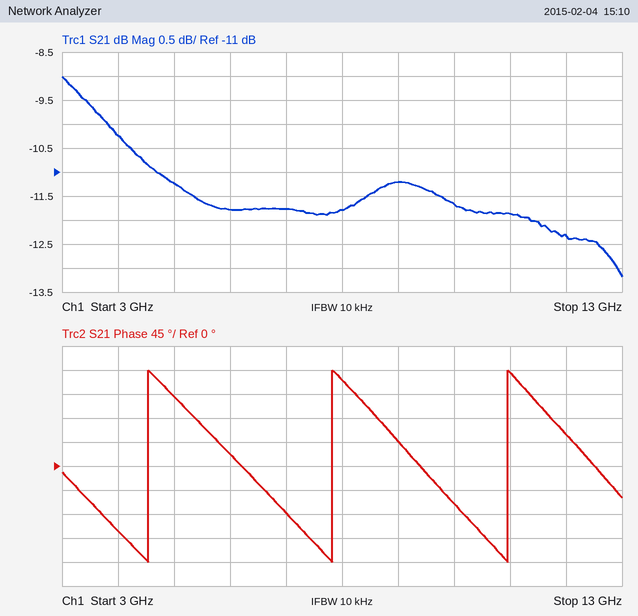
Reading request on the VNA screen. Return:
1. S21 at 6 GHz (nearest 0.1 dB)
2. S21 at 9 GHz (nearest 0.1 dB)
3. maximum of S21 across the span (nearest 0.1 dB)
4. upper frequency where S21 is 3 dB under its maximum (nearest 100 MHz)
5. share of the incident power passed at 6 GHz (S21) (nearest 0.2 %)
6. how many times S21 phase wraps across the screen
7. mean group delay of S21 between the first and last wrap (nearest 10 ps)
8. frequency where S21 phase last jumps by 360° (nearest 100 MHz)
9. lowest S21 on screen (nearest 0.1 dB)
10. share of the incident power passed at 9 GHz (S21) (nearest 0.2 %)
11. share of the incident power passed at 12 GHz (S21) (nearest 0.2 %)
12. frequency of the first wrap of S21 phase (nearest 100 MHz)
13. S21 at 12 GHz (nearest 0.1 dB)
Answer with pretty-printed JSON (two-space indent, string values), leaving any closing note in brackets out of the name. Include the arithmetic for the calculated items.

{
  "S21 at 6 GHz": "-11.8 dB",
  "S21 at 9 GHz": "-11.2 dB",
  "maximum of S21 across the span": "-9.0 dB",
  "upper frequency where S21 is 3 dB under its maximum": "11.4 GHz",
  "share of the incident power passed at 6 GHz (S21)": "10^(-11.8/10) ≈ 6.6 %",
  "how many times S21 phase wraps across the screen": "3",
  "mean group delay of S21 between the first and last wrap": "2 cycles / (11.0 GHz − 4.5 GHz) ≈ 308 ps, so 310 ps to the nearest 10 ps",
  "frequency where S21 phase last jumps by 360°": "11.0 GHz",
  "lowest S21 on screen": "-13.2 dB",
  "share of the incident power passed at 9 GHz (S21)": "10^(-11.2/10) ≈ 7.6 %",
  "share of the incident power passed at 12 GHz (S21)": "10^(-12.3/10) ≈ 5.89 %, so 5.8 % to the nearest 0.2 %",
  "frequency of the first wrap of S21 phase": "4.5 GHz",
  "S21 at 12 GHz": "-12.3 dB"
}
